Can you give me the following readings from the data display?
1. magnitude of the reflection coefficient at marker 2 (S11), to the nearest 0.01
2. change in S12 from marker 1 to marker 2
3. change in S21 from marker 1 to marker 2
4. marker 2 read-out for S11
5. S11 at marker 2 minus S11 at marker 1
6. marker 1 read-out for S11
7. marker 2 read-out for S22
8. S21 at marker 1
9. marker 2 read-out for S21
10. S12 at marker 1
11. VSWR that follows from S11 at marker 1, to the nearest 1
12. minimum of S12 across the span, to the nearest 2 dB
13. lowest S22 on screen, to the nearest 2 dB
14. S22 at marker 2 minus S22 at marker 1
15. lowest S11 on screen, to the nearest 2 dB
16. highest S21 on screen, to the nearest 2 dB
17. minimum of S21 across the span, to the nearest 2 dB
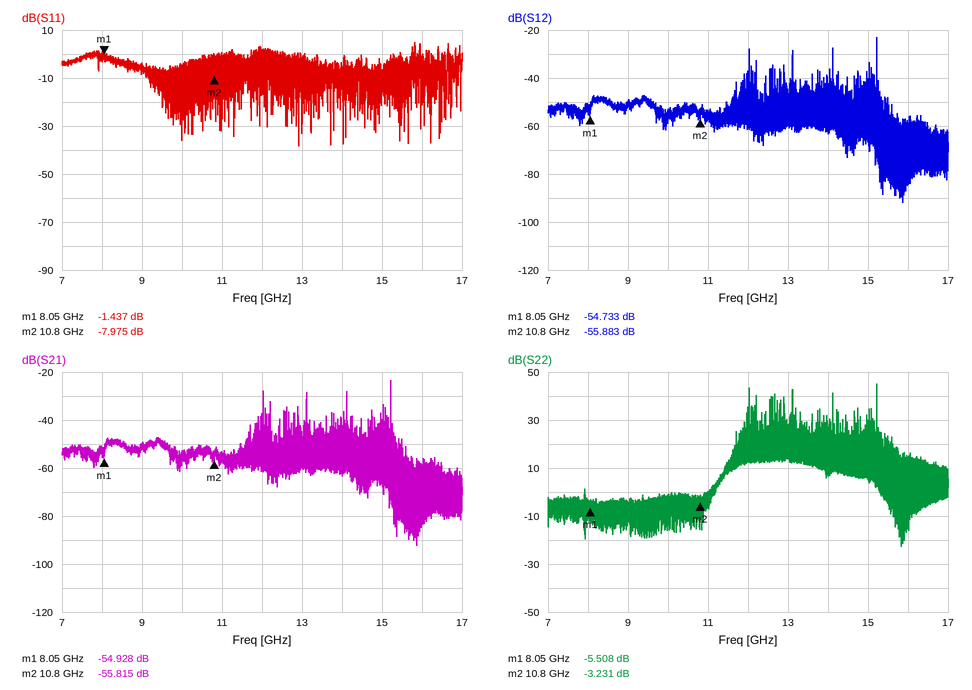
0.40
-1.150 dB
-0.887 dB
-7.975 dB
-6.538 dB
-1.437 dB
-3.231 dB
-54.928 dB
-55.815 dB
-54.733 dB
12
-92 dB
-22 dB
2.277 dB
-38 dB
-24 dB
-92 dB
